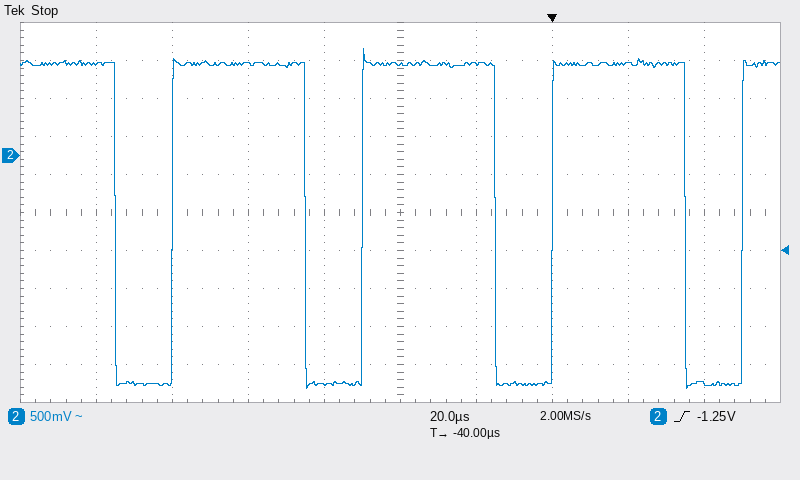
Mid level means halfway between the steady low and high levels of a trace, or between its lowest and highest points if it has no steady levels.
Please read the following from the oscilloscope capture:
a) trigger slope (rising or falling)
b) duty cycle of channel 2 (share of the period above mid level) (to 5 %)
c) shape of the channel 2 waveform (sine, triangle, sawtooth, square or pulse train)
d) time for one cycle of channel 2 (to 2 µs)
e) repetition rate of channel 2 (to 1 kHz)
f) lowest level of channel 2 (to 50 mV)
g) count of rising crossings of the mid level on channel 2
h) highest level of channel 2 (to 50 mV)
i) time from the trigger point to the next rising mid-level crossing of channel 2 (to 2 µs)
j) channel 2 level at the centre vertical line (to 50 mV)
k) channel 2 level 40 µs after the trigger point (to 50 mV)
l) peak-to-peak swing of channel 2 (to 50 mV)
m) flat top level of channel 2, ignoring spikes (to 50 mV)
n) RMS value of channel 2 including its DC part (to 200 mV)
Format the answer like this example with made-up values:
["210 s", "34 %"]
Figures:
["rising", "70 %", "pulse train", "50 µs", "20 kHz", "-3.05 V", "4", "1.40 V", "50 µs", "1.20 V", "-3.00 V", "4.45 V", "1.20 V", "2.0 V"]
